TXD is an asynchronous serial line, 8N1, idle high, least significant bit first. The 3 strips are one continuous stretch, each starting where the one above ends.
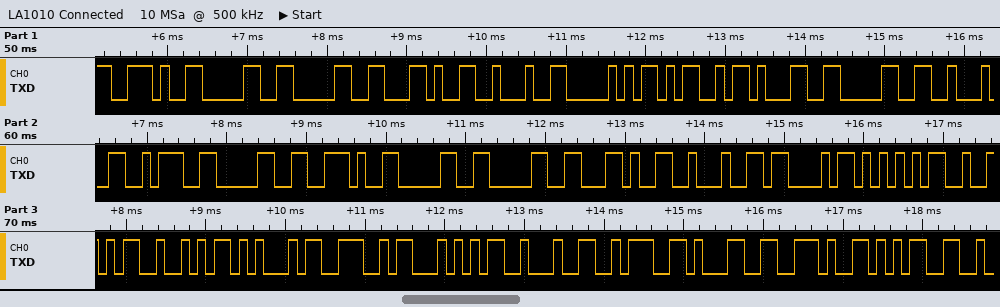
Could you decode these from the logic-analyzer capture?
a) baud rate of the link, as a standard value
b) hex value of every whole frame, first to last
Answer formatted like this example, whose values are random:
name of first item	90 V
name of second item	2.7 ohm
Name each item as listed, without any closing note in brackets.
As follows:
baud rate of the link, as a standard value	9600 baud
hex value of every whole frame, first to last	0x2E 0x30 0x30 0x2C 0x22 0x50 0x4D 0x31 0x30 0x22 0x3A 0x30 0x2E 0x30 0x30 0x2C 0x22 0x43 0x55 0x52 0x52 0x45 0x4E 0x54 0x22 0x3A 0x31 0x2E 0x35
